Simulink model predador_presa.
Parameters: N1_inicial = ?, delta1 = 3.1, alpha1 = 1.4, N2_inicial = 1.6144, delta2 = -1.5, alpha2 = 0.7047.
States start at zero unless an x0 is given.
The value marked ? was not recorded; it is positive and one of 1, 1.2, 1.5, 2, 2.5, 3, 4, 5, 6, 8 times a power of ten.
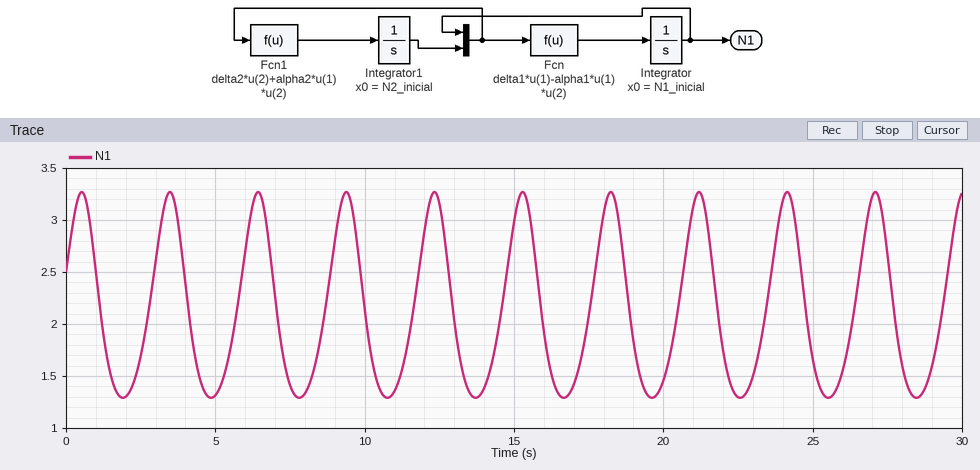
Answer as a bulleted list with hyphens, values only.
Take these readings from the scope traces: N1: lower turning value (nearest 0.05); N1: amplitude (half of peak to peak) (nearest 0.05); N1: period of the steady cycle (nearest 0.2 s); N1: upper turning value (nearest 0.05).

- 1.30
- 1.00
- 3.0 s
- 3.25
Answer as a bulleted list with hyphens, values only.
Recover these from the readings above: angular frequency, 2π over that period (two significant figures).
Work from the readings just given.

- 2.1 rad/s
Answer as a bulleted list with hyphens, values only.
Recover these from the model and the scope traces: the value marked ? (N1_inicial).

- 2.5
